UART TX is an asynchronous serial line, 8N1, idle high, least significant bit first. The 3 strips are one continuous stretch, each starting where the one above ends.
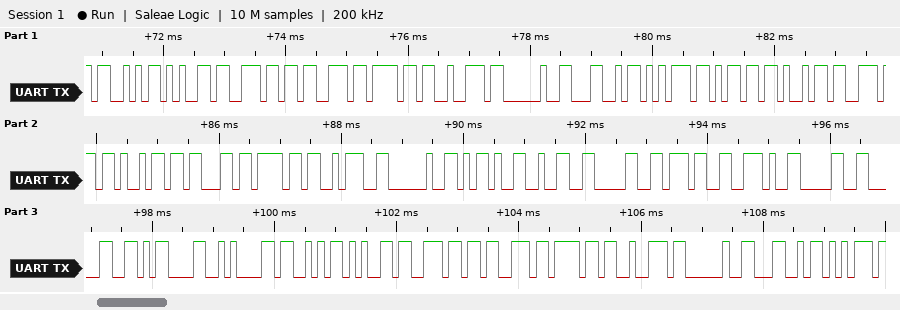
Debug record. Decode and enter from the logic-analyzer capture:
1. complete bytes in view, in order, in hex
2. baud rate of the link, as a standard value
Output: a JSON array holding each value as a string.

["0x53 0x65 0x6E 0x73 0x6F 0x72 0x20 0x4C 0x75 0x6D 0x69 0x6E 0x69 0x63 0x6F 0x3A 0x20 0x2D 0x32 0x30 0x37 0x2E 0x30 0x30 0x0D 0x0A 0x53 0x65 0x6E 0x73 0x6F 0x72 0x20 0x4C 0x75", "9600 baud"]
